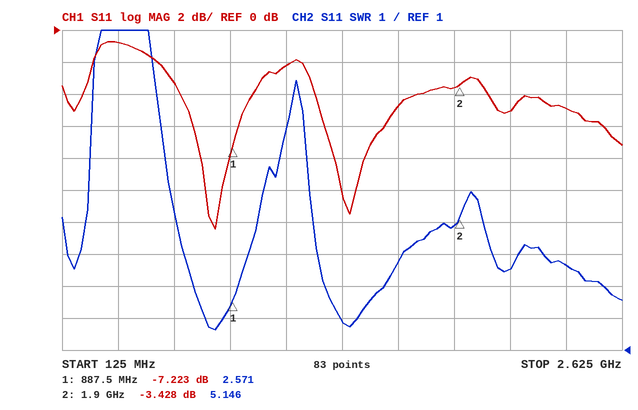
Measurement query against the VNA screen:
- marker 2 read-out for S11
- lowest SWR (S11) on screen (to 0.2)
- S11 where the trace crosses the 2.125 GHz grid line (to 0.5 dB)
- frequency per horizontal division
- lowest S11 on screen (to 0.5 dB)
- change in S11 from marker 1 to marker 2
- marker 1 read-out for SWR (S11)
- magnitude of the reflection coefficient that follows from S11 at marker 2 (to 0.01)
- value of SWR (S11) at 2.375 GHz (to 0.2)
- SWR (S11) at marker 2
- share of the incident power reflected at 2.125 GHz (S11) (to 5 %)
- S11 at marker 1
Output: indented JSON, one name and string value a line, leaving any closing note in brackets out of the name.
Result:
{
  "marker 2 read-out for S11": "-3.428 dB",
  "lowest SWR (S11) on screen": "1.6",
  "S11 where the trace crosses the 2.125 GHz grid line": "-5.0 dB",
  "frequency per horizontal division": "250 MHz",
  "lowest S11 on screen": "-12.5 dB",
  "change in S11 from marker 1 to marker 2": "3.795 dB",
  "marker 1 read-out for SWR": "2.571",
  "magnitude of the reflection coefficient that follows from S11 at marker 2": "0.67",
  "value of SWR (S11) at 2.375 GHz": "3.6",
  "SWR (S11) at marker 2": "5.146",
  "share of the incident power reflected at 2.125 GHz (S11)": "30 %",
  "S11 at marker 1": "-7.223 dB"
}
